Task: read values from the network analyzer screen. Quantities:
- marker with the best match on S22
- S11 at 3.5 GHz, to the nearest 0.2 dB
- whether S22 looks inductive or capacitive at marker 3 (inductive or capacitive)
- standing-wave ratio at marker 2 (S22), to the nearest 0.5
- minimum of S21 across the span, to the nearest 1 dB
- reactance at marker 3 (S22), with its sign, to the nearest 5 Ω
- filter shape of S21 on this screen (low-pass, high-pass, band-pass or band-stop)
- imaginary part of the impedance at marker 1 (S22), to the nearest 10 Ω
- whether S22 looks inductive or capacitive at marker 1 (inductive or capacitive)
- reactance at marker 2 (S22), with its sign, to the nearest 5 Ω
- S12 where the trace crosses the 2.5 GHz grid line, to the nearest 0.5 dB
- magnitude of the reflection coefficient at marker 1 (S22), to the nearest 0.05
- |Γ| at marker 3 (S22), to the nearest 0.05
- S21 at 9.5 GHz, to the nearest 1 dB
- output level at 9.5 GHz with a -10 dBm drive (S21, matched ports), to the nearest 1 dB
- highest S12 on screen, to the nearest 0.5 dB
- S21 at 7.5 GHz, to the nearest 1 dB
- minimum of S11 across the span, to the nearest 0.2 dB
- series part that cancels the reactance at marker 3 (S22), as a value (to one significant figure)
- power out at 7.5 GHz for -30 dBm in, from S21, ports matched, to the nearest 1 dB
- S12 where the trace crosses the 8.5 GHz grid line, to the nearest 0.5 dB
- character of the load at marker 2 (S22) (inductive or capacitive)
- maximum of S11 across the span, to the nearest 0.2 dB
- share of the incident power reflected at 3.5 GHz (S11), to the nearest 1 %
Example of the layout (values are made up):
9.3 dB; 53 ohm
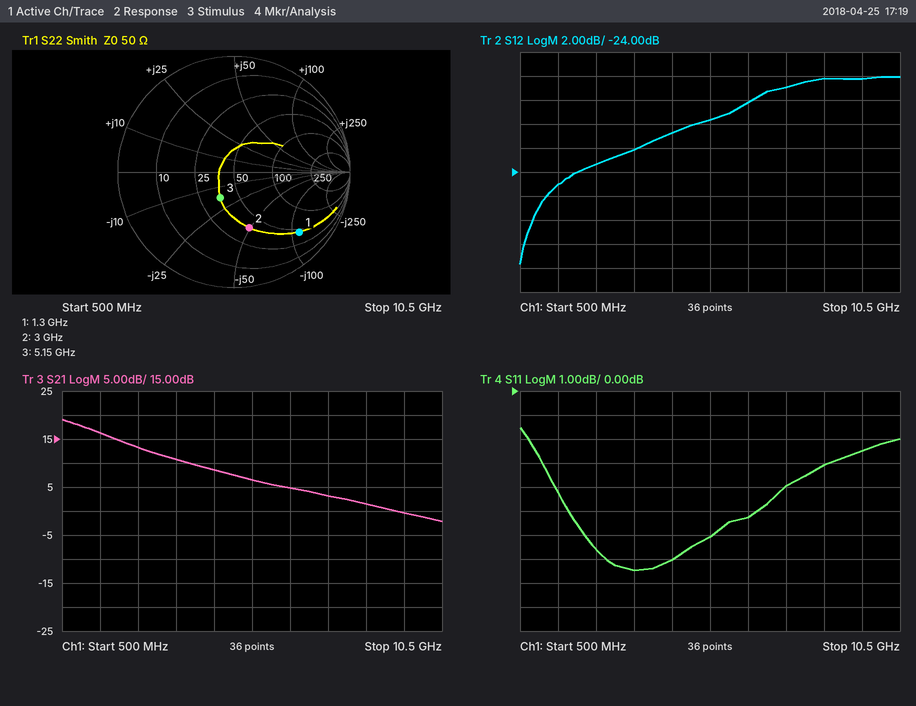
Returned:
marker 3; -7.4 dB; capacitive; 3.0; -2 dB; -15 Ω; low-pass; -110 Ω; capacitive; -50 Ω; -23.5 dB; 0.75; 0.25; 0 dB; -10 dBm; -16.0 dB; 3 dB; -7.4 dB; 500 pH; -27 dBm; -16.0 dB; capacitive; -1.6 dB; 18 %
